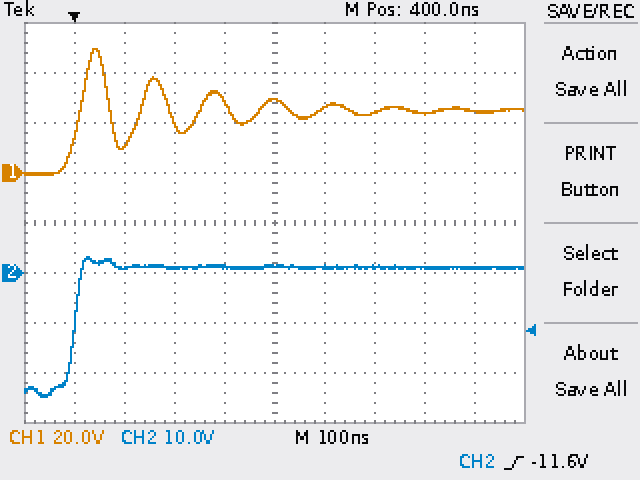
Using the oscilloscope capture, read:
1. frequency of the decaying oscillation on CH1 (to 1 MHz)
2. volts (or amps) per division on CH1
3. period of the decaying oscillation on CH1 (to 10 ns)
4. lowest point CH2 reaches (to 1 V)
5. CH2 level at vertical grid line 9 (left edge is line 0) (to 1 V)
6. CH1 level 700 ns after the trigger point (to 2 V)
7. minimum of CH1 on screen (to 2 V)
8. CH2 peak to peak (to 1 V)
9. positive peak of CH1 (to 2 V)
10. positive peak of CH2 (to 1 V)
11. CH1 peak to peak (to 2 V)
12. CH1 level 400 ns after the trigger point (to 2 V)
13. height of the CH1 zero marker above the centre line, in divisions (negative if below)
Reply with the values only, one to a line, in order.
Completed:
8 MHz
20 V
120 ns
-25 V
1 V
24 V
0 V
28 V
50 V
3 V
50 V
30 V
+1.0 div
